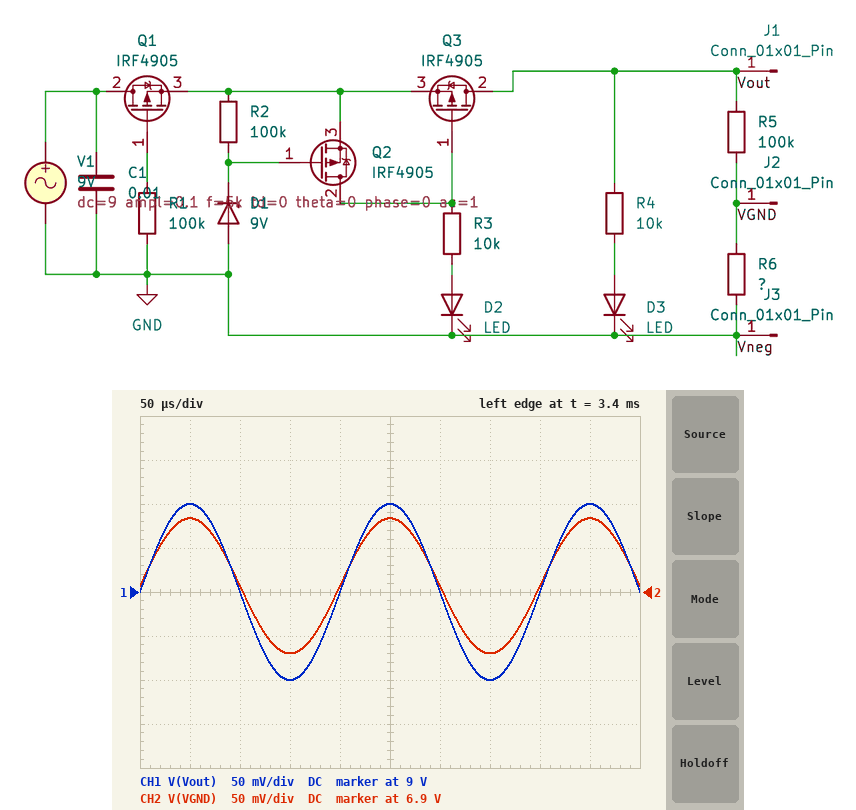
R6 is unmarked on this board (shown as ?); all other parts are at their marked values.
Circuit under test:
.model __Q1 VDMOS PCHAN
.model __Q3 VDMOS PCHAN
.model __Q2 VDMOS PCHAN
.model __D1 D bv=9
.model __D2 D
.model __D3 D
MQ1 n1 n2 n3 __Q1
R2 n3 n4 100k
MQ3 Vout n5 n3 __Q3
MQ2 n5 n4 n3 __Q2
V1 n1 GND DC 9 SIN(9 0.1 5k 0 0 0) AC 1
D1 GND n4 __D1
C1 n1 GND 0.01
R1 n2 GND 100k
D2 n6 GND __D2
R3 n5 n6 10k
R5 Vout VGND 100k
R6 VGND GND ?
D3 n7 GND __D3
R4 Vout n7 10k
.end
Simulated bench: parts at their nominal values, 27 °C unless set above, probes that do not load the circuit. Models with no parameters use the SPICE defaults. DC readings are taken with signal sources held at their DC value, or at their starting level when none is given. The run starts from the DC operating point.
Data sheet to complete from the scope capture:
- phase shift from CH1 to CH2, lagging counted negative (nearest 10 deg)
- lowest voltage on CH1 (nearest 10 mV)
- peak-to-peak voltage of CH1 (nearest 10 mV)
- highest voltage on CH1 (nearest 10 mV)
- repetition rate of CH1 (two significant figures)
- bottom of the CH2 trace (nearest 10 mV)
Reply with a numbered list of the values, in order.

1. 0 deg
2. 8.90 V
3. 200 mV
4. 9.10 V
5. 5.0 kHz
6. 6.83 V
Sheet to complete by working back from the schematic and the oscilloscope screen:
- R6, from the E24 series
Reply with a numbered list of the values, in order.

1. 330 kΩ
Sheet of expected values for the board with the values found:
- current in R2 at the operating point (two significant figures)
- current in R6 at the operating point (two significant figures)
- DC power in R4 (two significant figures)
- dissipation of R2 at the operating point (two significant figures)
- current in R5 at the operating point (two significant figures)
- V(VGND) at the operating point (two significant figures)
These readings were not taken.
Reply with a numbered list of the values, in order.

1. 1.7 µA
2. 21 µA
3. 7.0 mW
4. 270 nW
5. 21 µA
6. 6.9 V
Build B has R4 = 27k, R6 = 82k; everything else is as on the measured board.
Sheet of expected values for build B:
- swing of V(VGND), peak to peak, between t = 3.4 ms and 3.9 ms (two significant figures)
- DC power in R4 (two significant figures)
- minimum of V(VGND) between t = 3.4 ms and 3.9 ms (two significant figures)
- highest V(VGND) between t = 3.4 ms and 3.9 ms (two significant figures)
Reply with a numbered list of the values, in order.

1. 90 mV
2. 2.6 mW
3. 4.0 V
4. 4.1 V
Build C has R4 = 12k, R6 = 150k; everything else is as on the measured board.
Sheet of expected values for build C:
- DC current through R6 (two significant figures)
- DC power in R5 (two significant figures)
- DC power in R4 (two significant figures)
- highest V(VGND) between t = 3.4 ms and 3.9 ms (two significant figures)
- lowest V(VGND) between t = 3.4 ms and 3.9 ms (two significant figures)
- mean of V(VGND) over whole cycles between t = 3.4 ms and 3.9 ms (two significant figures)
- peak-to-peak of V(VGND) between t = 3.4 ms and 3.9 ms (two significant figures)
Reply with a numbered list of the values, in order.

1. 36 µA
2. 130 µW
3. 5.8 mW
4. 5.5 V
5. 5.3 V
6. 5.4 V
7. 120 mV
